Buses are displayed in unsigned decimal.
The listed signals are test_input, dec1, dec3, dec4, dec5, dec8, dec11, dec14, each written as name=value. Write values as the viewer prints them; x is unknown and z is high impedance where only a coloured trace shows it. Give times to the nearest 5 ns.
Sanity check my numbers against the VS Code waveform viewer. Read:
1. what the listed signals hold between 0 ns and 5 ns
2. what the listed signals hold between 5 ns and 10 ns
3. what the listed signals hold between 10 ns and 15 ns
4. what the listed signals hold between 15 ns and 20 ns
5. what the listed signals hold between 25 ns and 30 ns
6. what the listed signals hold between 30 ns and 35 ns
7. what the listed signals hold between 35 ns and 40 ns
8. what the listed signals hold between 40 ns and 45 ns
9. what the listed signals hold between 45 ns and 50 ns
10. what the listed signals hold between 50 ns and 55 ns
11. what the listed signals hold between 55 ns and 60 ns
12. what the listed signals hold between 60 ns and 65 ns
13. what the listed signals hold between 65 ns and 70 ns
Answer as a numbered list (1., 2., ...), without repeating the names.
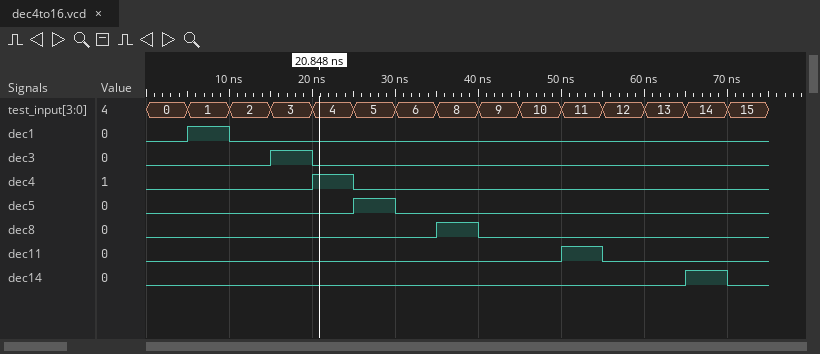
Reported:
1. test_input=0, dec1=0, dec3=0, dec4=0, dec5=0, dec8=0, dec11=0, dec14=0
2. test_input=1, dec1=1, dec3=0, dec4=0, dec5=0, dec8=0, dec11=0, dec14=0
3. test_input=2, dec1=0, dec3=0, dec4=0, dec5=0, dec8=0, dec11=0, dec14=0
4. test_input=3, dec1=0, dec3=1, dec4=0, dec5=0, dec8=0, dec11=0, dec14=0
5. test_input=5, dec1=0, dec3=0, dec4=0, dec5=1, dec8=0, dec11=0, dec14=0
6. test_input=6, dec1=0, dec3=0, dec4=0, dec5=0, dec8=0, dec11=0, dec14=0
7. test_input=8, dec1=0, dec3=0, dec4=0, dec5=0, dec8=1, dec11=0, dec14=0
8. test_input=9, dec1=0, dec3=0, dec4=0, dec5=0, dec8=0, dec11=0, dec14=0
9. test_input=10, dec1=0, dec3=0, dec4=0, dec5=0, dec8=0, dec11=0, dec14=0
10. test_input=11, dec1=0, dec3=0, dec4=0, dec5=0, dec8=0, dec11=1, dec14=0
11. test_input=12, dec1=0, dec3=0, dec4=0, dec5=0, dec8=0, dec11=0, dec14=0
12. test_input=13, dec1=0, dec3=0, dec4=0, dec5=0, dec8=0, dec11=0, dec14=0
13. test_input=14, dec1=0, dec3=0, dec4=0, dec5=0, dec8=0, dec11=0, dec14=1
